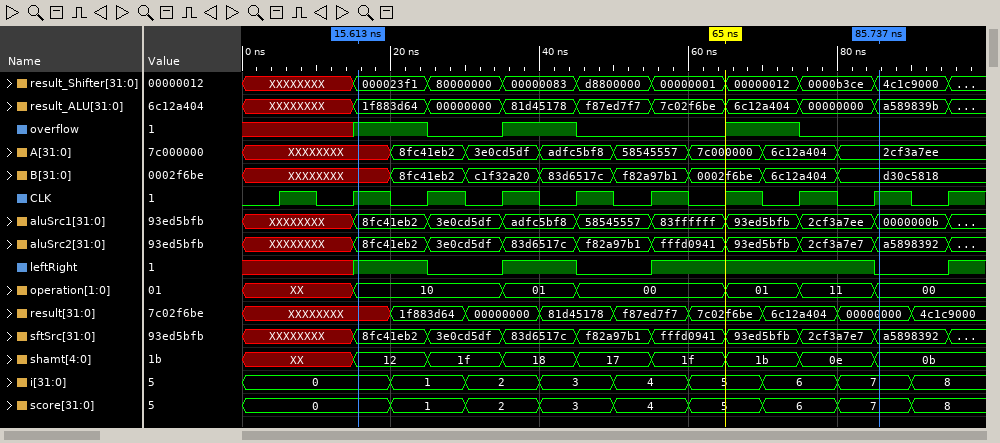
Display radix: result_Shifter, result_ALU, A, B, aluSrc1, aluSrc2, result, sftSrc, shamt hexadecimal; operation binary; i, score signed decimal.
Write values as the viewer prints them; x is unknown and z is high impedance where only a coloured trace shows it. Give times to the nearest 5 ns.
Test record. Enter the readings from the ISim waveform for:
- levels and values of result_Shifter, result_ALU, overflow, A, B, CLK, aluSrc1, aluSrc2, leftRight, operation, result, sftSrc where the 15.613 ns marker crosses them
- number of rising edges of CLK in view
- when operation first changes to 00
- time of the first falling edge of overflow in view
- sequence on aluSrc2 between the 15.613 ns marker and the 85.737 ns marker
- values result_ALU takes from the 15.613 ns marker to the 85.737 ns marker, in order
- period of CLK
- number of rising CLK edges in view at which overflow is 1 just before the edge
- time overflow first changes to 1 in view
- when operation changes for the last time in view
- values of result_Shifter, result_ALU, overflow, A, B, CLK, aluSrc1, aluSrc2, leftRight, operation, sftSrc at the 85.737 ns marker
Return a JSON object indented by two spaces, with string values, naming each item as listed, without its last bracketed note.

{
  "levels and values of result_Shifter, result_ALU, overflow, A, B, CLK, aluSrc1, aluSrc2, leftRight, operation, result, sftSrc where the 15.613 ns marker crosses them": "result_Shifter=000023f1, result_ALU=1f883d64, overflow=1, A=XXXXXXXX, B=XXXXXXXX, CLK=1, aluSrc1=8fc41eb2, aluSrc2=8fc41eb2, leftRight=1, operation=10, result=XXXXXXXX, sftSrc=8fc41eb2",
  "number of rising edges of CLK in view": "10",
  "when operation first changes to 00": "45 ns",
  "time of the first falling edge of overflow in view": "25 ns",
  "sequence on aluSrc2 between the 15.613 ns marker and the 85.737 ns marker": "8fc41eb2, 3e0cd5df, 83d6517c, f82a97b1, fffd0941, 93ed5bfb, 2cf3a7e7, a5898392",
  "values result_ALU takes from the 15.613 ns marker to the 85.737 ns marker, in order": "1f883d64, 00000000, 81d45178, f87ed7f7, 7c02f6be, 6c12a404, 00000000, a589839b",
  "period of CLK": "10 ns",
  "number of rising CLK edges in view at which overflow is 1 just before the edge": "3",
  "time overflow first changes to 1 in view": "15 ns",
  "when operation changes for the last time in view": "85 ns",
  "values of result_Shifter, result_ALU, overflow, A, B, CLK, aluSrc1, aluSrc2, leftRight, operation, sftSrc at the 85.737 ns marker": "result_Shifter=4c1c9000, result_ALU=a589839b, overflow=0, A=2cf3a7ee, B=d30c5818, CLK=1, aluSrc1=0000000b, aluSrc2=a5898392, leftRight=0, operation=00, sftSrc=a5898392"
}
